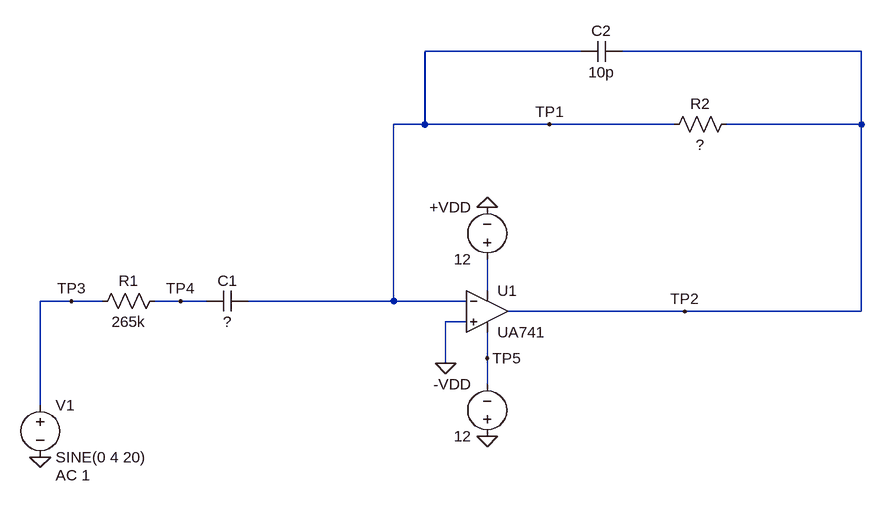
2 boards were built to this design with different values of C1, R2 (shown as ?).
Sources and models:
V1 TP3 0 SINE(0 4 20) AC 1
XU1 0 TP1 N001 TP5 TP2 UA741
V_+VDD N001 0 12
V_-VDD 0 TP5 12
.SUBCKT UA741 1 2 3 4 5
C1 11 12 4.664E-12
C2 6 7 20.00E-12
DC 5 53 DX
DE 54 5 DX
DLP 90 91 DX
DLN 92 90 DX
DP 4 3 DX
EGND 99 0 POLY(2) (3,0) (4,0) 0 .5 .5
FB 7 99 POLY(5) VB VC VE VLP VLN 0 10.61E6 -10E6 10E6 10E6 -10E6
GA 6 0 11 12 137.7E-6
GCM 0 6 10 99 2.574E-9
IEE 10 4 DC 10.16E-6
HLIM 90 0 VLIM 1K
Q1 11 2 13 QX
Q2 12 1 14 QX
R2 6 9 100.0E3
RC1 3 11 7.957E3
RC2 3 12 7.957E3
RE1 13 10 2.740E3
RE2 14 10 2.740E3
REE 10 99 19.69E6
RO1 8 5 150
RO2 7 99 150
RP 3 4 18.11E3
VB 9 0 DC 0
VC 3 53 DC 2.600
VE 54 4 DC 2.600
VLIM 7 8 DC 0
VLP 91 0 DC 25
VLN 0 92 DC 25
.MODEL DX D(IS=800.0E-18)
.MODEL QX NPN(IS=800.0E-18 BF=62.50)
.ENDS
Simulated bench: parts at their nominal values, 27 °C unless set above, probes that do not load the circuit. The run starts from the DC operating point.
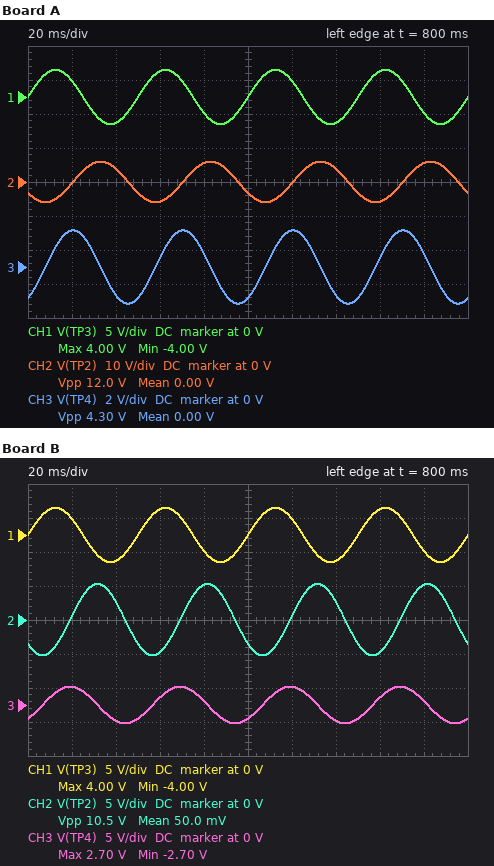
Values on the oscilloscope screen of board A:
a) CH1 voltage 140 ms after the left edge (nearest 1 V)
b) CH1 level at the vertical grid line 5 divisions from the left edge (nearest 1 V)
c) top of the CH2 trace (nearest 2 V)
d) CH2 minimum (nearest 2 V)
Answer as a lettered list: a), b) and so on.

a) -4 V
b) 0 V
c) 6 V
d) -6 V
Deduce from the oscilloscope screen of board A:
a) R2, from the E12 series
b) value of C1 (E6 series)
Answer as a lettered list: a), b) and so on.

a) 470 kΩ
b) 47 nF
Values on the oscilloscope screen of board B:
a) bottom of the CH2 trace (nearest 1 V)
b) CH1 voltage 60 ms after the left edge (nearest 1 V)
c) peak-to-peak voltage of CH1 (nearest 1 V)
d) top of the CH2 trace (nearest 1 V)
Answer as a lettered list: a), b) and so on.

a) -5 V
b) 4 V
c) 8 V
d) 5 V
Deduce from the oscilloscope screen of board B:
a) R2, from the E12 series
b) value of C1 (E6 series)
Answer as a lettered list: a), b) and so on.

a) 470 kΩ
b) 33 nF
